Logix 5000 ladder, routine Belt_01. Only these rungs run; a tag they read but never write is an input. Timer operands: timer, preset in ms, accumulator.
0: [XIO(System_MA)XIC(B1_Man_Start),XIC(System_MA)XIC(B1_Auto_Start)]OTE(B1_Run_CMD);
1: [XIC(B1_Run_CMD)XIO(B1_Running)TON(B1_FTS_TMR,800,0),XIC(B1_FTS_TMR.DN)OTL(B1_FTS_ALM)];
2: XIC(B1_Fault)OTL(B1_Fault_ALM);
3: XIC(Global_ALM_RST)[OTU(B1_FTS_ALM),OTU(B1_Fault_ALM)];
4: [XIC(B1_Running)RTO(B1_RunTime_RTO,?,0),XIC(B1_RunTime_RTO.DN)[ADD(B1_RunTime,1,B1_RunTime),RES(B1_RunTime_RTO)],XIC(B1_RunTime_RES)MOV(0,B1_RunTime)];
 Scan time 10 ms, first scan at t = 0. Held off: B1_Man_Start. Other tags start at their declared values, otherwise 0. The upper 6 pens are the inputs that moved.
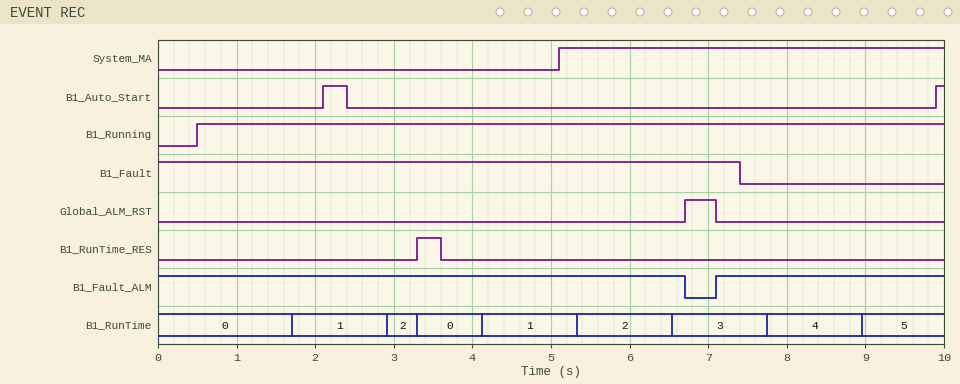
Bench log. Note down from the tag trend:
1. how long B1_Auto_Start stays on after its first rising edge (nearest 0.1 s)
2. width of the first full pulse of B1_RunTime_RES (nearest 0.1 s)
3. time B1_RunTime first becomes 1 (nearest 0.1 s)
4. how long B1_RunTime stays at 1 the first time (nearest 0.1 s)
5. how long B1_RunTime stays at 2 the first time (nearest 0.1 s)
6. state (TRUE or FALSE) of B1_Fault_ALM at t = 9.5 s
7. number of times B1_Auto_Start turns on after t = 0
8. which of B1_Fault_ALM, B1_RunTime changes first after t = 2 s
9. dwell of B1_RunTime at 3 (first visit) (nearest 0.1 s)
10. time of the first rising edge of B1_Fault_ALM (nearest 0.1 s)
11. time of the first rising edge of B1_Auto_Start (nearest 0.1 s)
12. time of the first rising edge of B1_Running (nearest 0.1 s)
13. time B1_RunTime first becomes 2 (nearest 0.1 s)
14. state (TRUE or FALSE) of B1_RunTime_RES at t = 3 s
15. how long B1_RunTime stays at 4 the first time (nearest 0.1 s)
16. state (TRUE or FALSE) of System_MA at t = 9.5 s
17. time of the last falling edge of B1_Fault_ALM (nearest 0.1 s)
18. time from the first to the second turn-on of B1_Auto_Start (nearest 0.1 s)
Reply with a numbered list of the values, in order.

1. 0.3 s
2. 0.3 s
3. 1.7 s
4. 1.2 s
5. 0.4 s
6. TRUE
7. 2
8. B1_RunTime
9. 1.2 s
10. 7.1 s
11. 2.1 s
12. 0.5 s
13. 2.9 s
14. FALSE
15. 1.2 s
16. TRUE
17. 6.7 s
18. 7.8 s
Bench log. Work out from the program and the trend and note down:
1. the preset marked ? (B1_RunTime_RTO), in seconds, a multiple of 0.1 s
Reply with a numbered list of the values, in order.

1. 1.2 s
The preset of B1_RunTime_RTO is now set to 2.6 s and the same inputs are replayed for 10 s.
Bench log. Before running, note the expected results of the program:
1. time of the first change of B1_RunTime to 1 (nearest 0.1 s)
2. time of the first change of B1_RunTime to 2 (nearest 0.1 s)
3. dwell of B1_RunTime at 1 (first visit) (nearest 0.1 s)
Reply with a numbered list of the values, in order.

1. 3.1 s
2. 8.3 s
3. 0.2 s
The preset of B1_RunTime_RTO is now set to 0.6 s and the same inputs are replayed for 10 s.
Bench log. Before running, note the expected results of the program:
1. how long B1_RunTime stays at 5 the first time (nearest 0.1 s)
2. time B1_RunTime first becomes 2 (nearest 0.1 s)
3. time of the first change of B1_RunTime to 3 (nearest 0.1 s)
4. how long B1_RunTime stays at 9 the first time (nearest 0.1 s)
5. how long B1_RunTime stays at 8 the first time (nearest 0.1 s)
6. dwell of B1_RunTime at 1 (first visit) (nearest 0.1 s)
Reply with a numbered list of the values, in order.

1. 0.6 s
2. 1.7 s
3. 2.3 s
4. 0.6 s
5. 0.6 s
6. 0.6 s
